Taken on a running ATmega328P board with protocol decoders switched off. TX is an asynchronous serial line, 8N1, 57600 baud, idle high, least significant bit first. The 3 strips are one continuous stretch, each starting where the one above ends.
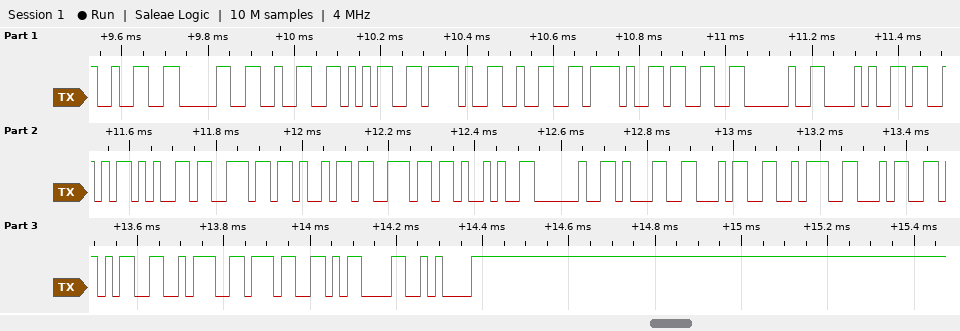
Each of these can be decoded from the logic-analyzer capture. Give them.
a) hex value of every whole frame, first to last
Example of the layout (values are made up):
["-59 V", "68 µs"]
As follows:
["32 30 32 35 2F 32 2F 33 20 28 53 65 6E 69 6E 29 20 31 34 3A 34 35 3A 37 0D 0A"]
